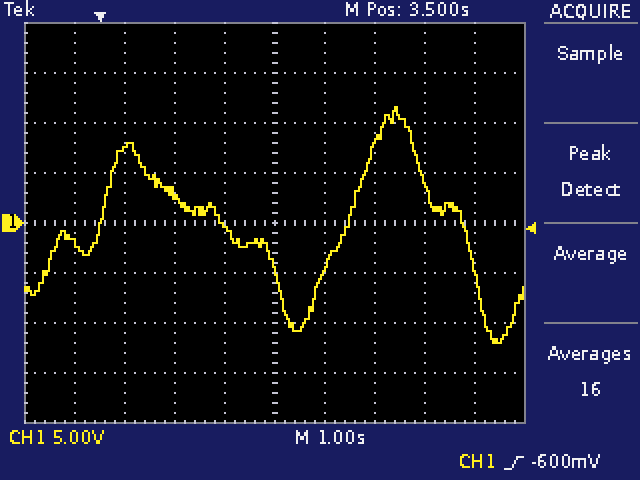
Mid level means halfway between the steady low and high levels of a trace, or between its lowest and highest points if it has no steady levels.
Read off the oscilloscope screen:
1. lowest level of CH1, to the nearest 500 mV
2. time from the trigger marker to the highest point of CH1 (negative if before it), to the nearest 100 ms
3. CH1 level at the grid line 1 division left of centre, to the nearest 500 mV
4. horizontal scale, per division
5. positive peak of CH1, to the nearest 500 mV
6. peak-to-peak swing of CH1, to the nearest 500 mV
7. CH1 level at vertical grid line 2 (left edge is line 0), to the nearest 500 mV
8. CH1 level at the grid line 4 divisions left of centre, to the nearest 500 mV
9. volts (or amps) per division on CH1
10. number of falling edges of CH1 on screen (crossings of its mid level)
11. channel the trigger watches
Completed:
-12.0 V
+5.9 s
-500 mV
1 s
11.5 V
23.5 V
7.5 V
-2.0 V
5 V
2
CH1
